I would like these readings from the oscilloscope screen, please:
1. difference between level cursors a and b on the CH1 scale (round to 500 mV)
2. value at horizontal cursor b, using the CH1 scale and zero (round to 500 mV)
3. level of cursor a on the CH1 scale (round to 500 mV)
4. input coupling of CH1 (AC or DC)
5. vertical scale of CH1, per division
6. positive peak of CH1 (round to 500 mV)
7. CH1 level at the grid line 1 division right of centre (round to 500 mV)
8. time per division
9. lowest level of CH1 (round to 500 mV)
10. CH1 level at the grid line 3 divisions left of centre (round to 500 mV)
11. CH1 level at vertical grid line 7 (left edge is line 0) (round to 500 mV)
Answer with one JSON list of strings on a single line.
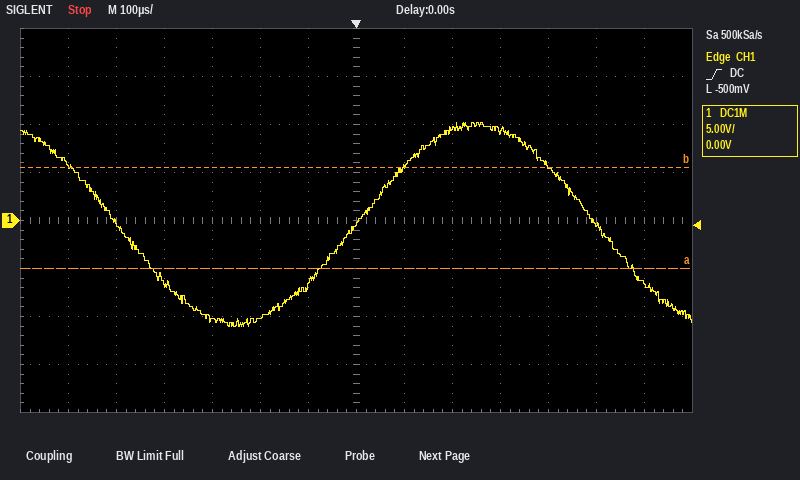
["10.5 V", "5.5 V", "-5.0 V", "DC", "5 V", "10.0 V", "5.5 V", "100 µs", "-11.0 V", "-10.5 V", "-500 mV"]
